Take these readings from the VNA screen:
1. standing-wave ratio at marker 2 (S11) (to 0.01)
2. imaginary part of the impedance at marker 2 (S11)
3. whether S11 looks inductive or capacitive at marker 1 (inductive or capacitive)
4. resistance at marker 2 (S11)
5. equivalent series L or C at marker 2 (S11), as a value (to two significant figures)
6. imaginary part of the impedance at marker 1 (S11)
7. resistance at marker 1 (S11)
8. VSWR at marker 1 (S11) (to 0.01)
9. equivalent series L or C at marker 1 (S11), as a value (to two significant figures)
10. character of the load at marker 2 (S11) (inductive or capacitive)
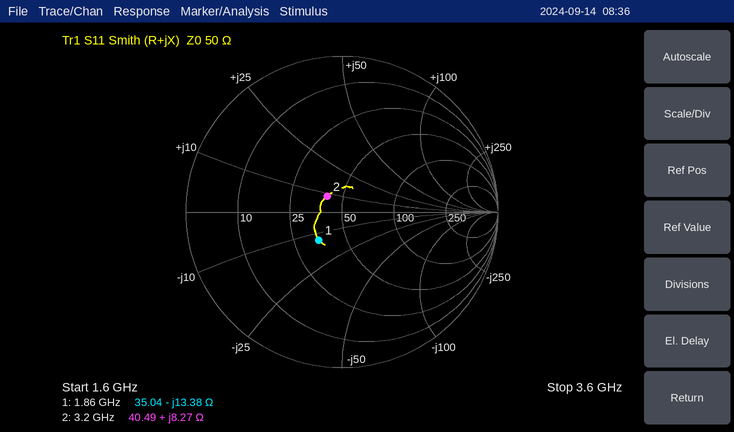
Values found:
1.32
+8.27 Ω
capacitive
40.49 Ω
410 pH
-13.38 Ω
35.04 Ω
1.61
6.4 pF
inductive
